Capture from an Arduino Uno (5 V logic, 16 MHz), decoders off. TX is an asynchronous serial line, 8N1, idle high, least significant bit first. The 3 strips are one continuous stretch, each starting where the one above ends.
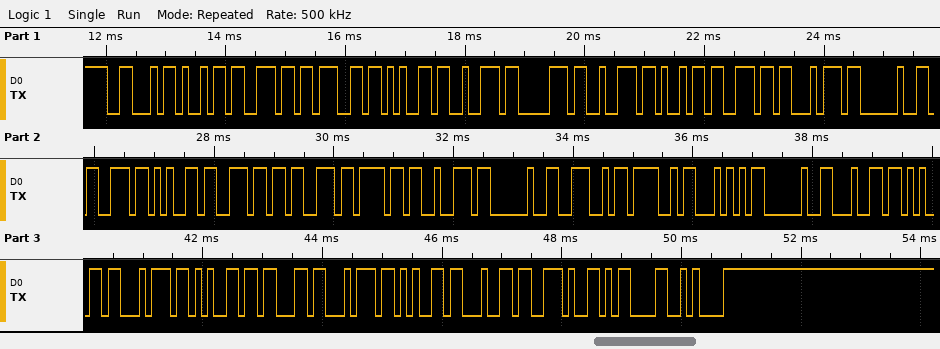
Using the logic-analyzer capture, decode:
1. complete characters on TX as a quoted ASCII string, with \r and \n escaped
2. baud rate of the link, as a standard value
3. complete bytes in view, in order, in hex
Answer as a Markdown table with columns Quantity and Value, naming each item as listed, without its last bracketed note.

| Quantity | Value |
|---|---|
| complete characters on TX as a quoted ASCII string, with \r and \n escaped | "Fingerprint sensor NOT detected.\r\n" |
| baud rate of the link, as a standard value | 9600 baud |
| complete bytes in view, in order, in hex | 0x46 0x69 0x6E 0x67 0x65 0x72 0x70 0x72 0x69 0x6E 0x74 0x20 0x73 0x65 0x6E 0x73 0x6F 0x72 0x20 0x4E 0x4F 0x54 0x20 0x64 0x65 0x74 0x65 0x63 0x74 0x65 0x64 0x2E 0x0D 0x0A |
